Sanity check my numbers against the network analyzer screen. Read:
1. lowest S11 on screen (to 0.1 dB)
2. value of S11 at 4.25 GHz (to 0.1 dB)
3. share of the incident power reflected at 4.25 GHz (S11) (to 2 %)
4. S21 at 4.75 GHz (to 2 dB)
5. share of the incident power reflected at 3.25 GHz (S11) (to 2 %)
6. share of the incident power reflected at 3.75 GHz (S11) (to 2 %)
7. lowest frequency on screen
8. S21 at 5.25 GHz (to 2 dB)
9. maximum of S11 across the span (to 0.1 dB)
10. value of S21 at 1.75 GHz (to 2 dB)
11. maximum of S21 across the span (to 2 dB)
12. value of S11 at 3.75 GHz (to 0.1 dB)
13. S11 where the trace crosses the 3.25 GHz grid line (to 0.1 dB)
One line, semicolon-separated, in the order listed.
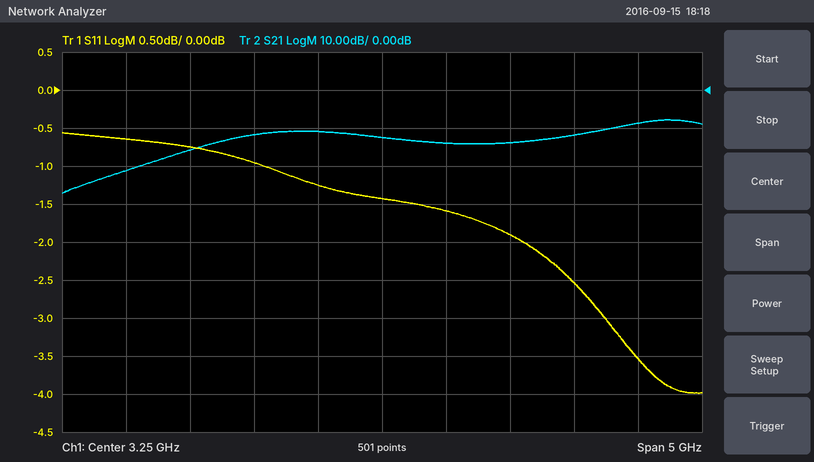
-4.0 dB; -1.9 dB; 64 %; -12 dB; 72 %; 70 %; 750 MHz; -8 dB; -0.6 dB; -16 dB; -8 dB; -1.6 dB; -1.4 dB
